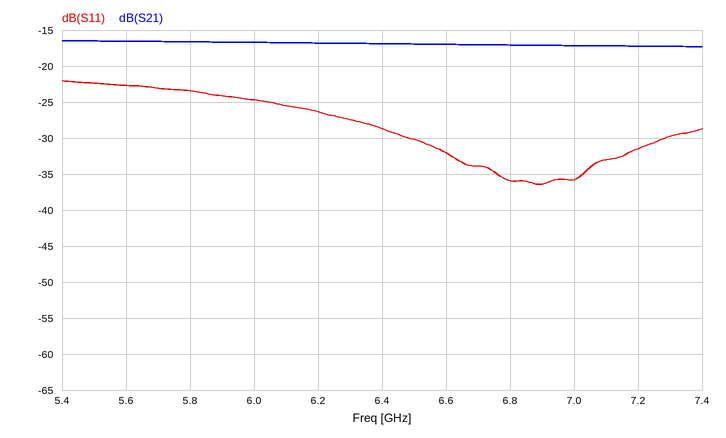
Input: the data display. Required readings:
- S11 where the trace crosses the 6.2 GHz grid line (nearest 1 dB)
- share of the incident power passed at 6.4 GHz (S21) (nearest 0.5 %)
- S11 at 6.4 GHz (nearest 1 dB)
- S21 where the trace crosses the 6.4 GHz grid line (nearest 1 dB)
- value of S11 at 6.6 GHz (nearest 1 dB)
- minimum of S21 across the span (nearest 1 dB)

-26 dB
2.0 %
-29 dB
-17 dB
-32 dB
-17 dB
